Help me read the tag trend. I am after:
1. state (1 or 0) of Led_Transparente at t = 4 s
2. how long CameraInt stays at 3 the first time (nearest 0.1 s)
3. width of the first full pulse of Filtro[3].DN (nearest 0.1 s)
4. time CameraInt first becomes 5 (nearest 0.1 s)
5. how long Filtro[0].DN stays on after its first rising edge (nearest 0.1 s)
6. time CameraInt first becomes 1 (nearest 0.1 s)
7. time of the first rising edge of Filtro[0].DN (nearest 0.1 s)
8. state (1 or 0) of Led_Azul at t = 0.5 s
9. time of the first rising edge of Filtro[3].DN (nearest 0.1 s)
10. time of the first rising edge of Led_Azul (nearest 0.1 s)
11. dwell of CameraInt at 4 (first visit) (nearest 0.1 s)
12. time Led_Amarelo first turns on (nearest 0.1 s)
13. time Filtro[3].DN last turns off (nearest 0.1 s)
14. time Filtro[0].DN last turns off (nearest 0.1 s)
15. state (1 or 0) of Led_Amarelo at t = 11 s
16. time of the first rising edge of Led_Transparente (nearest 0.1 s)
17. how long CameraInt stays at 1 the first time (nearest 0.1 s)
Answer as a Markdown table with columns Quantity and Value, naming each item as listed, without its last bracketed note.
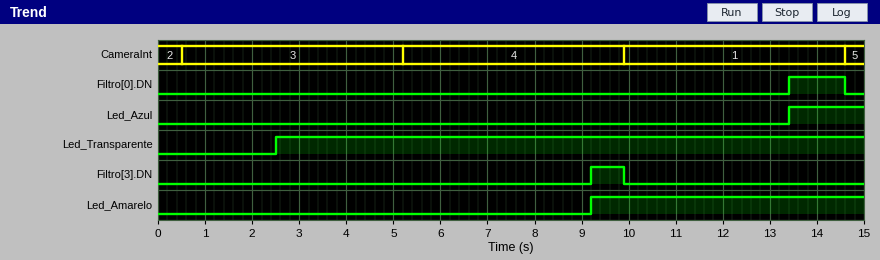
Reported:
| Quantity | Value |
|---|---|
| state (1 or 0) of Led_Transparente at t = 4 s | 1 |
| how long CameraInt stays at 3 the first time | 4.7 s |
| width of the first full pulse of Filtro[3].DN | 0.7 s |
| time CameraInt first becomes 5 | 14.6 s |
| how long Filtro[0].DN stays on after its first rising edge | 1.2 s |
| time CameraInt first becomes 1 | 9.9 s |
| time of the first rising edge of Filtro[0].DN | 13.4 s |
| state (1 or 0) of Led_Azul at t = 0.5 s | 0 |
| time of the first rising edge of Filtro[3].DN | 9.2 s |
| time of the first rising edge of Led_Azul | 13.4 s |
| dwell of CameraInt at 4 (first visit) | 4.7 s |
| time Led_Amarelo first turns on | 9.2 s |
| time Filtro[3].DN last turns off | 9.9 s |
| time Filtro[0].DN last turns off | 14.6 s |
| state (1 or 0) of Led_Amarelo at t = 11 s | 1 |
| time of the first rising edge of Led_Transparente | 2.5 s |
| how long CameraInt stays at 1 the first time | 4.7 s |
